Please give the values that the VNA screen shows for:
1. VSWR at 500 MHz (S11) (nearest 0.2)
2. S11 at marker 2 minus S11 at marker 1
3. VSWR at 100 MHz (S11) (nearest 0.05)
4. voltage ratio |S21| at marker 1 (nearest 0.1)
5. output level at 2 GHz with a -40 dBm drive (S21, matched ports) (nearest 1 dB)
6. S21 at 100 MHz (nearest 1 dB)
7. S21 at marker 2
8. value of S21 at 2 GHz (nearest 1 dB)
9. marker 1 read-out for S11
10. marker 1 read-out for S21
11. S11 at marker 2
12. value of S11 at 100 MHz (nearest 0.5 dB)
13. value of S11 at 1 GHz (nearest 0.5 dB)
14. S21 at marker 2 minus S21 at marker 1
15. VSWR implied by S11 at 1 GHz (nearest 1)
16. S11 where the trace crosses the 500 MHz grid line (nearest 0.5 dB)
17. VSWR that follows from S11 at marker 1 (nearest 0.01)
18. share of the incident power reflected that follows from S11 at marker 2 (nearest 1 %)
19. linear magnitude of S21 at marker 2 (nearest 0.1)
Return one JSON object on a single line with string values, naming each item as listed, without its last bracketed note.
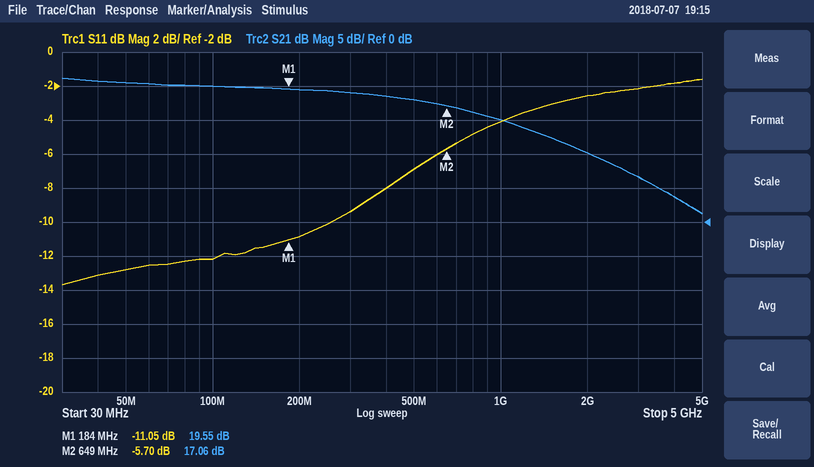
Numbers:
{"VSWR at 500 MHz (S11)": "2.6", "S11 at marker 2 minus S11 at marker 1": "5.35 dB", "VSWR at 100 MHz (S11)": "1.65", "voltage ratio |S21| at marker 1": "9.5", "output level at 2 GHz with a -40 dBm drive (S21, matched ports)": "-30 dBm", "S21 at 100 MHz": "20 dB", "S21 at marker 2": "17.06 dB", "value of S21 at 2 GHz": "10 dB", "marker 1 read-out for S11": "-11.05 dB", "marker 1 read-out for S21": "19.55 dB", "S11 at marker 2": "-5.70 dB", "value of S11 at 100 MHz": "-12.0 dB", "value of S11 at 1 GHz": "-4.0 dB", "S21 at marker 2 minus S21 at marker 1": "-2.49 dB", "VSWR implied by S11 at 1 GHz": "4", "S11 where the trace crosses the 500 MHz grid line": "-7.0 dB", "VSWR that follows from S11 at marker 1": "1.78", "share of the incident power reflected that follows from S11 at marker 2": "27 %", "linear magnitude of S21 at marker 2": "7.1"}
